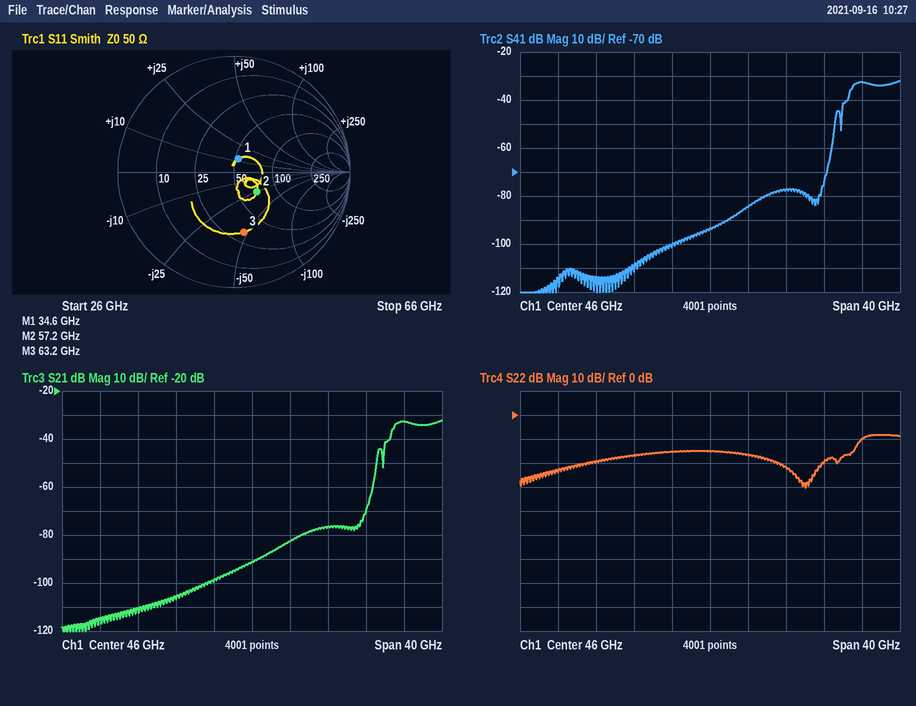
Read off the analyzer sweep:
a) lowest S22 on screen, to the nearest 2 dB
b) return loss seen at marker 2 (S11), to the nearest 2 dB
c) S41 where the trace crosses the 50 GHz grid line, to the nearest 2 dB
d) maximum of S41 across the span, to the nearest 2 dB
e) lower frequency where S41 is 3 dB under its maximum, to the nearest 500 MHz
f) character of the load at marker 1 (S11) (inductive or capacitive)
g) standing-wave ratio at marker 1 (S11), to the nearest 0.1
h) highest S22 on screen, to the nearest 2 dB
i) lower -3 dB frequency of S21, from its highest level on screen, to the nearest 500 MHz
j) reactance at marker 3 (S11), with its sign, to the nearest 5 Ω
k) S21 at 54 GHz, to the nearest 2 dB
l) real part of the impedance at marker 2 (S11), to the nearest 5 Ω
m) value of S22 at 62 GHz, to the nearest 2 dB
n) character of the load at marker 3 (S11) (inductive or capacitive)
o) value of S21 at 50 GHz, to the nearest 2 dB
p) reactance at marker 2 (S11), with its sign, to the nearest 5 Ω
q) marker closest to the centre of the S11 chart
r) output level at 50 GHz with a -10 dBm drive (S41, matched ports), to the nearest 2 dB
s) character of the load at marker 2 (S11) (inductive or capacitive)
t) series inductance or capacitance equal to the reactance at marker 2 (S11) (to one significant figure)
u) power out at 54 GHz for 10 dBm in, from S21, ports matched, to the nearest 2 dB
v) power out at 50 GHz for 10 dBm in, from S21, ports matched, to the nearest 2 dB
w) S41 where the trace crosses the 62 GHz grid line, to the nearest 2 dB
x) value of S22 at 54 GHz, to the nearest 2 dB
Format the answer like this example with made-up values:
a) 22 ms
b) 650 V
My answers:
a) -30 dB
b) 12 dB
c) -84 dB
d) -32 dB
e) 61.0 GHz
f) inductive
g) 1.3
h) -8 dB
i) 61.0 GHz
j) -45 Ω
k) -76 dB
l) 70 Ω
m) -10 dB
n) capacitive
o) -82 dB
p) -25 Ω
q) marker 1
r) -94 dBm
s) capacitive
t) 100 fF
u) -66 dBm
v) -72 dBm
w) -32 dB
x) -22 dB
